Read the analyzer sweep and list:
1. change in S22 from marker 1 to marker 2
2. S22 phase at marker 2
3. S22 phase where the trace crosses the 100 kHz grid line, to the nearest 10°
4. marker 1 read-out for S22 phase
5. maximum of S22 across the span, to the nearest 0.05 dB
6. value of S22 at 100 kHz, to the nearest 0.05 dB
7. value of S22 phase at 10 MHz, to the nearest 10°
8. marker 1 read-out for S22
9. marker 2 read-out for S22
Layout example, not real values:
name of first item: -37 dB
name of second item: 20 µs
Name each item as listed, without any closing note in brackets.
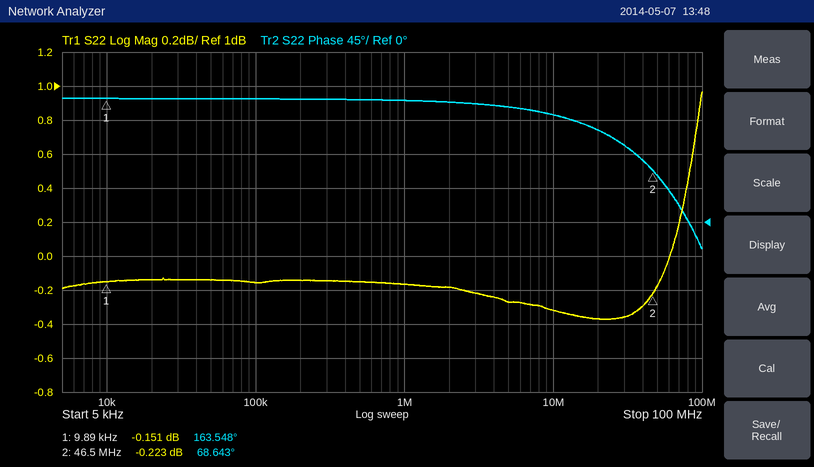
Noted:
change in S22 from marker 1 to marker 2: -0.072 dB
S22 phase at marker 2: 68.643°
S22 phase where the trace crosses the 100 kHz grid line, to the nearest 10°: 160°
marker 1 read-out for S22 phase: 163.548°
maximum of S22 across the span, to the nearest 0.05 dB: 0.95 dB
value of S22 at 100 kHz, to the nearest 0.05 dB: -0.15 dB
value of S22 phase at 10 MHz, to the nearest 10°: 140°
marker 1 read-out for S22: -0.151 dB
marker 2 read-out for S22: -0.223 dB
